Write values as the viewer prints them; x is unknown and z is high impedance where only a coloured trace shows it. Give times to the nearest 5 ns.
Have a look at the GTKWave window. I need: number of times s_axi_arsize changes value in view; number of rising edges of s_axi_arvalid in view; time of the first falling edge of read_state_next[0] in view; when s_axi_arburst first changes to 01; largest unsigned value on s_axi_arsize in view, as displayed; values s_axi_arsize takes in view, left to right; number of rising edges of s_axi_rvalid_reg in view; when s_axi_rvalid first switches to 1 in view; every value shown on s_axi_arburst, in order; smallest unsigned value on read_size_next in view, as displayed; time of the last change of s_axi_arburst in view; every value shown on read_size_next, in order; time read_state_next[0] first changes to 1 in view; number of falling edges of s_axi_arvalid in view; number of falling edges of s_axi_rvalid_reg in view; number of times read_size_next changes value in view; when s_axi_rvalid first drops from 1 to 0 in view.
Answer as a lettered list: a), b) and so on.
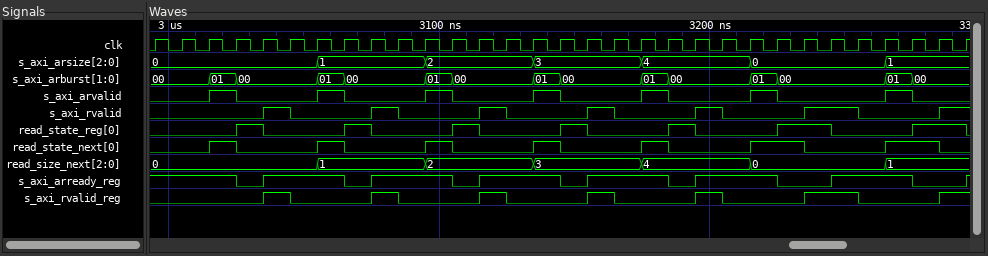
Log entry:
a) 6
b) 7
c) 3025 ns
d) 3015 ns
e) 4
f) 0, 1, 2, 3, 4, 0, 1
g) 7
h) 3035 ns
i) 00, 01, 00, 01, 00, 01, 00, 01, 00, 01, 00, 01, 00, 01, 00
j) 0
k) 3275 ns
l) 0, 1, 2, 3, 4, 0, 1
m) 3015 ns
n) 7
o) 6
p) 6
q) 3045 ns
